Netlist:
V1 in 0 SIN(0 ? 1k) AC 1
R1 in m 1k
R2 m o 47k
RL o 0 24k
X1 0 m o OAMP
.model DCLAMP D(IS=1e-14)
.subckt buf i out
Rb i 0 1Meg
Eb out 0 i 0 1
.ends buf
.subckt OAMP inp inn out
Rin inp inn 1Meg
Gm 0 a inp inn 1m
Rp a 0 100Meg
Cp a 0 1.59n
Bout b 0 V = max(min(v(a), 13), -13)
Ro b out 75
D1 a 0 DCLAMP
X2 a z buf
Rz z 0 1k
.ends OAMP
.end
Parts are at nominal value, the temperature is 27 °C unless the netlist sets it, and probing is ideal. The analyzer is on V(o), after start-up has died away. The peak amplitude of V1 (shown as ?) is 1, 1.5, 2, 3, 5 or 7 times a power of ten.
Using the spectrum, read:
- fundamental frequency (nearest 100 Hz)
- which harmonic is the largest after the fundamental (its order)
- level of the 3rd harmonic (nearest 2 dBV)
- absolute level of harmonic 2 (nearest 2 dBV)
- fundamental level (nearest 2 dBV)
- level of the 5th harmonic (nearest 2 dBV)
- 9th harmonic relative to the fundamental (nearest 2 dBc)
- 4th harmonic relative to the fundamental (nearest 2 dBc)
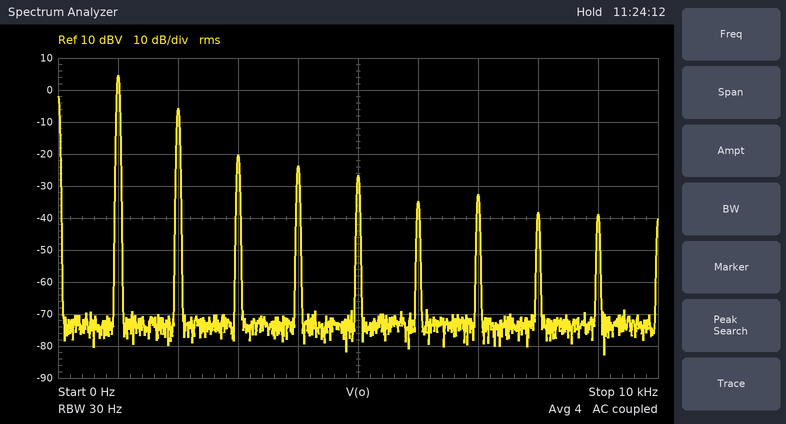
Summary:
1.0 kHz
2
-20 dBV
-6 dBV
4 dBV
-26 dBV
-44 dBc
-28 dBc
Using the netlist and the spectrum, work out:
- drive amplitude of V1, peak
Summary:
100 mV
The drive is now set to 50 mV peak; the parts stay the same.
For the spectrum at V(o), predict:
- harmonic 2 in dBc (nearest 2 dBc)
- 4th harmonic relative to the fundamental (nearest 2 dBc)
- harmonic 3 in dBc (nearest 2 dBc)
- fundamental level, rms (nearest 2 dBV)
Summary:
-12 dBc
-34 dBc
-24 dBc
0 dBV
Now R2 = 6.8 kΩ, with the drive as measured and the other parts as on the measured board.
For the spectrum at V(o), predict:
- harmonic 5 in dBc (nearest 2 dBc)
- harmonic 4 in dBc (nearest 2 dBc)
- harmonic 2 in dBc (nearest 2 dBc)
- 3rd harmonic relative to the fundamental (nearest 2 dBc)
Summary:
-40 dBc
-34 dBc
-26 dBc
-28 dBc
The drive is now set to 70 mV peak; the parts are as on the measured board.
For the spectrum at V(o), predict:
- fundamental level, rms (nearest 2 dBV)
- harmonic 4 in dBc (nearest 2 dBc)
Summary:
2 dBV
-30 dBc
